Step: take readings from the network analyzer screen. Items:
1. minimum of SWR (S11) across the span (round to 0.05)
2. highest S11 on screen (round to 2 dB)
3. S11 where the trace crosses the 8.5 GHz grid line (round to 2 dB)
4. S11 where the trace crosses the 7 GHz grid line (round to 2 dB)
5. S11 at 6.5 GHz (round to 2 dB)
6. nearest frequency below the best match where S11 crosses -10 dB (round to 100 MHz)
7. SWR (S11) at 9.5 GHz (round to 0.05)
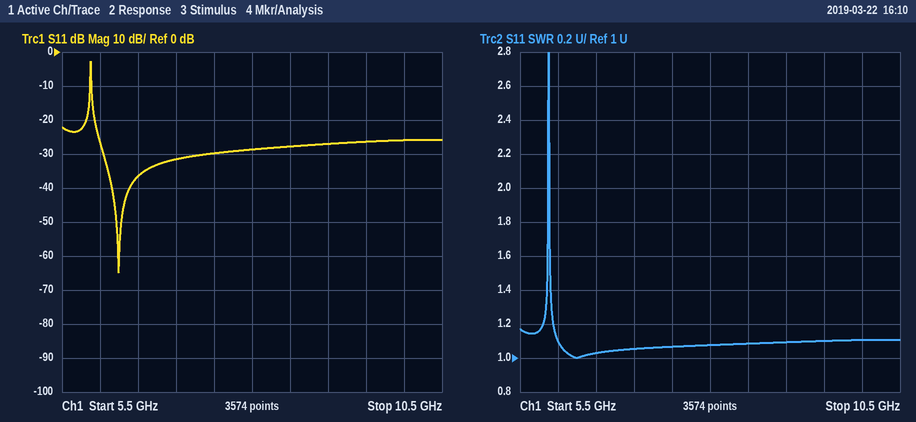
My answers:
1.00
-2 dB
-28 dB
-32 dB
-36 dB
5.9 GHz
1.10
